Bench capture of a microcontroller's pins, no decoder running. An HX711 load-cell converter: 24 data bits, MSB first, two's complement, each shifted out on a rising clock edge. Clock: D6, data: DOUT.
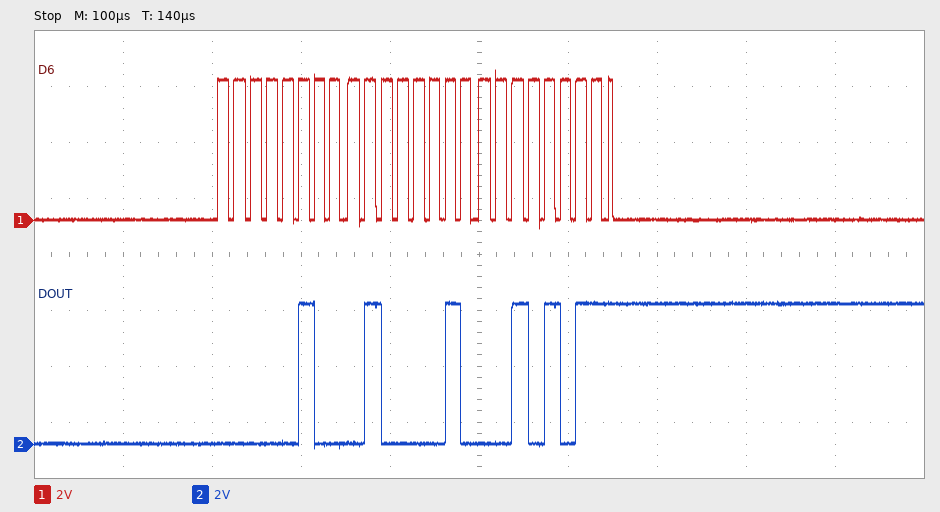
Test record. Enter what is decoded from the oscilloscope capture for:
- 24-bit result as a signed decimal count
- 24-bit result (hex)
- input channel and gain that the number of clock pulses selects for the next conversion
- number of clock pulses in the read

279083
0x04422B
channel A, gain 128
25
